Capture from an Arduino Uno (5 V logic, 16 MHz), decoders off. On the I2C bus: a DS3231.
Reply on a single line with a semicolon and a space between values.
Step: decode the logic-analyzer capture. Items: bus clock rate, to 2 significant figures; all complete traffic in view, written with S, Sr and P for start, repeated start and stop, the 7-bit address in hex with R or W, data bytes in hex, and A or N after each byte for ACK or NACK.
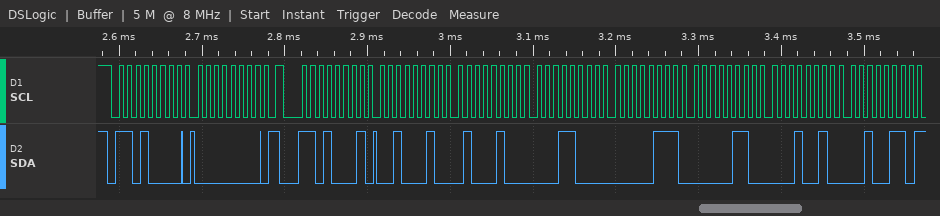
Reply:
100 kHz; S 68W A 00 A Sr 68R A 22 A 44 A 18 A 07 A 06 A 12 A 26 N
